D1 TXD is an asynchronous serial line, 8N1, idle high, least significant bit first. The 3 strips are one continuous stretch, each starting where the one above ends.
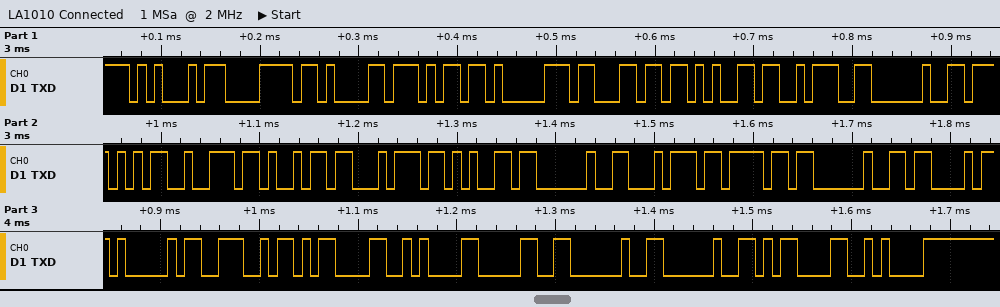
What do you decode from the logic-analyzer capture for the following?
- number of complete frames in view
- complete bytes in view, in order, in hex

28
45 78 61 6D 70 6C 65 3A 20 57 72 69 74 65 20 74 6F 20 43 41 4E 0D 0A 30 20 20 0D 0A
